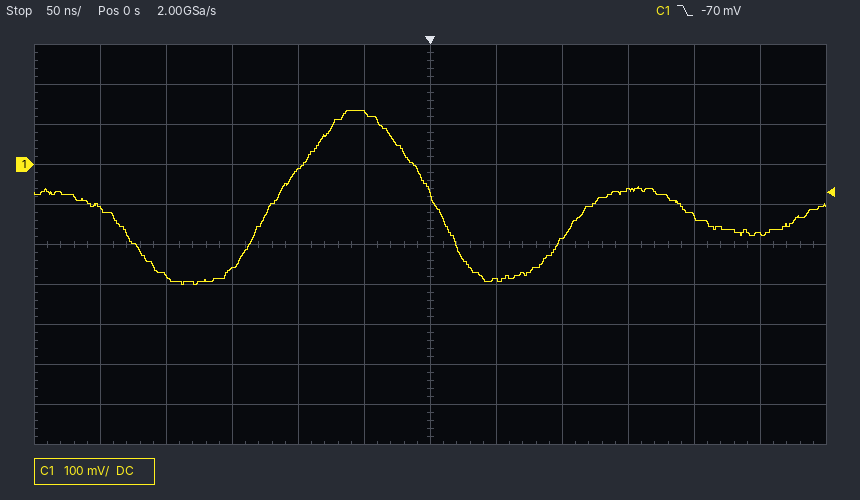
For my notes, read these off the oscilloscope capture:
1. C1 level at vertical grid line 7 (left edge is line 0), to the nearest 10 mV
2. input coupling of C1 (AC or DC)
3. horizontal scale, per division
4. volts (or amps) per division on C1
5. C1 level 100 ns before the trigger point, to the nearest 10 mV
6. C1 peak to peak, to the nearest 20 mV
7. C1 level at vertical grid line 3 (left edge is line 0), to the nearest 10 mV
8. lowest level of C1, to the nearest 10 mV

-290 mV
DC
50 ns
100 mV
-10 mV
440 mV
-260 mV
-300 mV
